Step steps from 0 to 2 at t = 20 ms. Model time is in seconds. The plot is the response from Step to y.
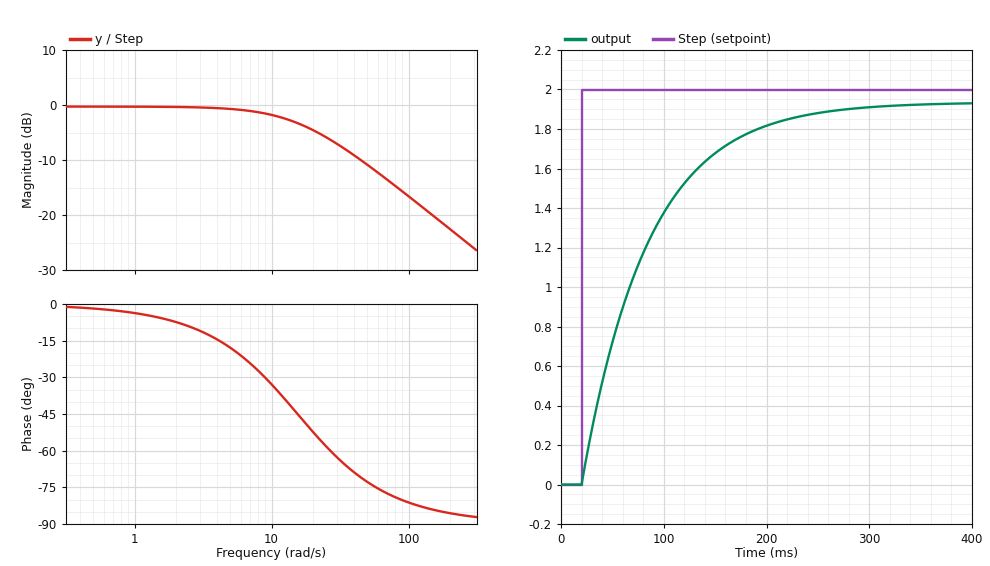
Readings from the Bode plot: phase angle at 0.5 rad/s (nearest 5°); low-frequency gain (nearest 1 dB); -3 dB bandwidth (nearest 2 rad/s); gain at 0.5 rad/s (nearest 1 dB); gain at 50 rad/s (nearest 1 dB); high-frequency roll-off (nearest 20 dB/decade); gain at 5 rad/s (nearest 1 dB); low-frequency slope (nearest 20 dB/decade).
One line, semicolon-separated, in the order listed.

0°; 0 dB; 16 rad/s; 0 dB; -11 dB; -20 dB/decade; -1 dB; 0 dB/decade
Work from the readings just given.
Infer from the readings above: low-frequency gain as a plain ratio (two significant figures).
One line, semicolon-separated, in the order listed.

1.0
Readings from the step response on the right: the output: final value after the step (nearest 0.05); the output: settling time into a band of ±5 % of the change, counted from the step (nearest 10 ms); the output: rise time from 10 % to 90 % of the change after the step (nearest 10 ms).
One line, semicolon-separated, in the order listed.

1.95; 190 ms; 140 ms
